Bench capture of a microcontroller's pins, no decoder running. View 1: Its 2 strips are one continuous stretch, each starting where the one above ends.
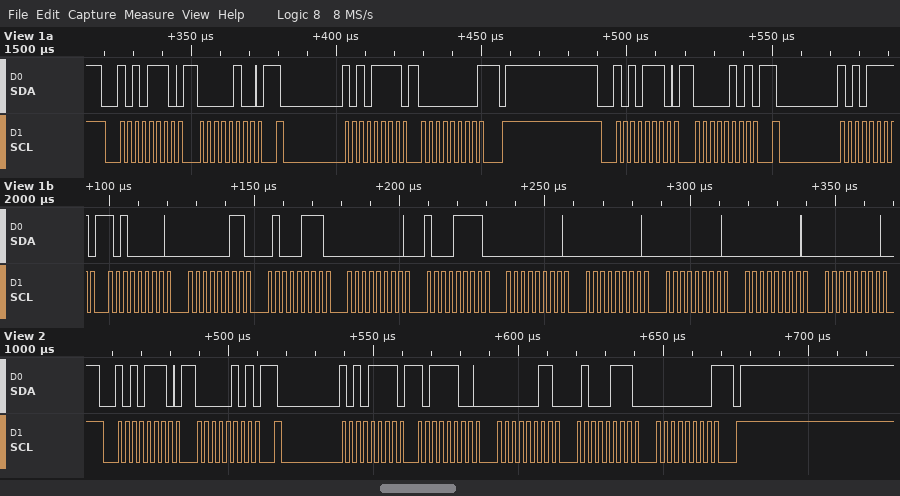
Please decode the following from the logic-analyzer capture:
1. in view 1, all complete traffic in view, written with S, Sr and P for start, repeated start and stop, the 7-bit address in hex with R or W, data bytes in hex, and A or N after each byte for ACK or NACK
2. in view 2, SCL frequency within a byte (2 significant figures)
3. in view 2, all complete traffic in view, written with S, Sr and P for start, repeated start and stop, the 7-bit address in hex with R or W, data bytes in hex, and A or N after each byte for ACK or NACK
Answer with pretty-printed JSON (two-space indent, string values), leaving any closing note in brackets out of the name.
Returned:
{
  "in view 1, all complete traffic in view, written with S, Sr and P for start, repeated start and stop, the 7-bit address in hex with R or W, data bytes in hex, and A or N after each byte for ACK or NACK": "S 57W A 04 A Sr 57R A 00 N P S 57W A 05 A Sr 57R A A0 A 03 A 47 A 00 A 8F A 00 A 00 A 00 A 00 A 00 A",
  "in view 2, SCL frequency within a byte": "400 kHz",
  "in view 2, all complete traffic in view, written with S, Sr and P for start, repeated start and stop, the 7-bit address in hex with R or W, data bytes in hex, and A or N after each byte for ACK or NACK": "S 57W A 05 A Sr 57R A BC A 03 A 47 A 00 N P"
}
